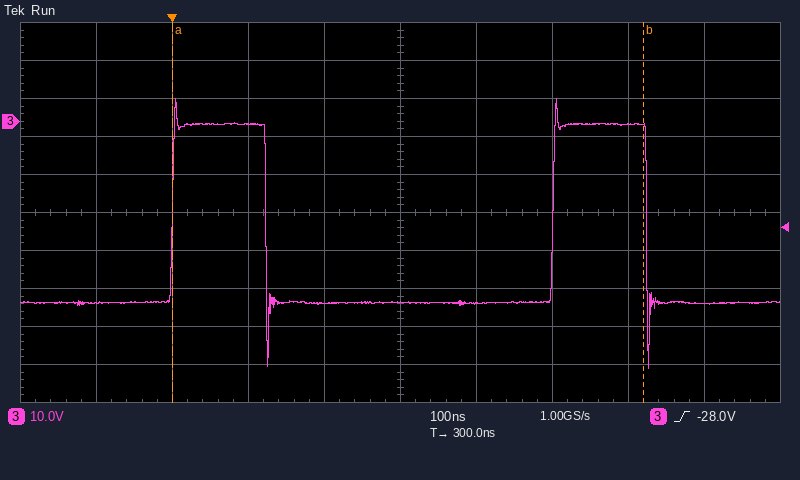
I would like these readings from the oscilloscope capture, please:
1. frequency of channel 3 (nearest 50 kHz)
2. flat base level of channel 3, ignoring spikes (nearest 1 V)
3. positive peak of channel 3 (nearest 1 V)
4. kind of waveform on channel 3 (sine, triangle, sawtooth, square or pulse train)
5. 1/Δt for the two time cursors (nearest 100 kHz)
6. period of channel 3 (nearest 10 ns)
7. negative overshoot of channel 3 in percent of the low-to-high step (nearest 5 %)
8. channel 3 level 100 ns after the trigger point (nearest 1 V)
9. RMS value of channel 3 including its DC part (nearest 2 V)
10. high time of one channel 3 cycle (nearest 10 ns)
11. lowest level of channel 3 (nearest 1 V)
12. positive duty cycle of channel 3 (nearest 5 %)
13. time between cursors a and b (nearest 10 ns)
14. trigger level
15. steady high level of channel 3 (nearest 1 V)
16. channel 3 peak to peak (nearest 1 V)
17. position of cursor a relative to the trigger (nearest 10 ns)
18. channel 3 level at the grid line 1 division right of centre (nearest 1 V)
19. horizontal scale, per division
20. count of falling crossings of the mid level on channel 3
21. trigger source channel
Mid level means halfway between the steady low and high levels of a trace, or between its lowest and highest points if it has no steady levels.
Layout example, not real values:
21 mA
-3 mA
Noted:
2.00 MHz
-48 V
6 V
pulse train
1.6 MHz
500 ns
35 %
-1 V
42 V
120 ns
-65 V
25 %
620 ns
-28.0 V
-1 V
71 V
0 ns
-48 V
100 ns
2
channel 3
